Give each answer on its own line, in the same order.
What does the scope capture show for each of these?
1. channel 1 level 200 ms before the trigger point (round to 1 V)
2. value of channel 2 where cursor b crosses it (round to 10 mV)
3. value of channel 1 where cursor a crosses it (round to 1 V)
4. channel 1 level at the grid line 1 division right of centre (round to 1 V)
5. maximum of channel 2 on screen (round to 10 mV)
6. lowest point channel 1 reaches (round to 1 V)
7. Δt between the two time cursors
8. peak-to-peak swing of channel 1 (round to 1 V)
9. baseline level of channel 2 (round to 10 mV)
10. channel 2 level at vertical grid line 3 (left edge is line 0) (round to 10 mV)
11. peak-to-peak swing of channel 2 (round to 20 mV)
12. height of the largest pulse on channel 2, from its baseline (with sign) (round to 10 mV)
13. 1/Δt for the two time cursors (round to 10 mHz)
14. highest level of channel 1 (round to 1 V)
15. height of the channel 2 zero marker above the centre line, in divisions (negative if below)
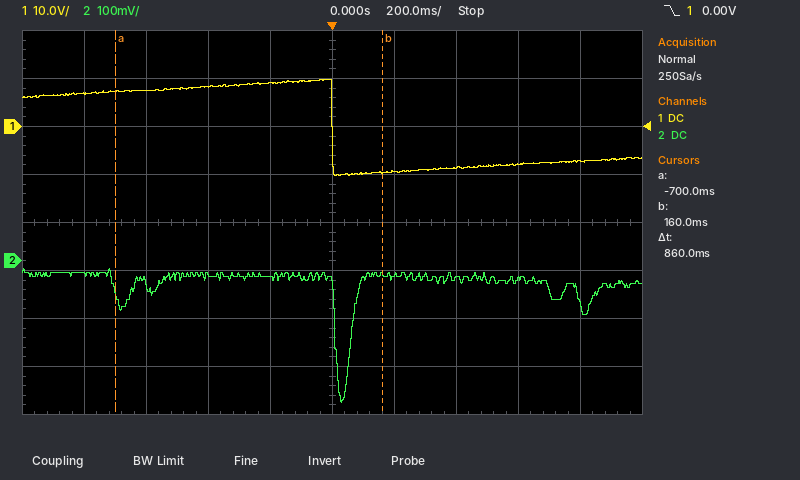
9 V
-30 mV
7 V
-9 V
-20 mV
-10 V
860 ms
20 V
-30 mV
-30 mV
280 mV
-260 mV
1.16 Hz
10 V
-0.8 div
